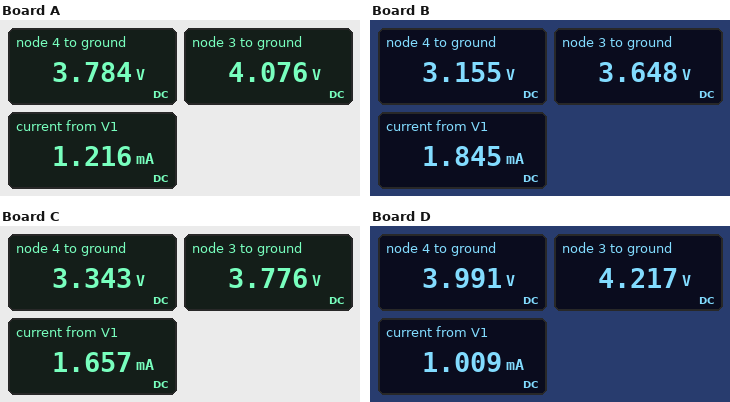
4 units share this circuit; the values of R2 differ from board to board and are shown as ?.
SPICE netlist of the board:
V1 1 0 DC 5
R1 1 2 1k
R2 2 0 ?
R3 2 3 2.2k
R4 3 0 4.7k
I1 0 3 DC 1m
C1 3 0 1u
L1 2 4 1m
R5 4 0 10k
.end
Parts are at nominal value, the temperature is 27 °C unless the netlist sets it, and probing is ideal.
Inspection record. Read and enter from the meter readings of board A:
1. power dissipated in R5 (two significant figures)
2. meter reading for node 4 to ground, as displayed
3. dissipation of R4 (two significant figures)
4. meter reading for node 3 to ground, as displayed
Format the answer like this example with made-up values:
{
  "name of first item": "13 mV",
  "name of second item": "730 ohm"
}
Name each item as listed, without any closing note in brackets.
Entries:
{
  "power dissipated in R5": "1.4 mW",
  "meter reading for node 4 to ground, as displayed": "3.784 V",
  "dissipation of R4": "3.5 mW",
  "meter reading for node 3 to ground, as displayed": "4.076 V"
}
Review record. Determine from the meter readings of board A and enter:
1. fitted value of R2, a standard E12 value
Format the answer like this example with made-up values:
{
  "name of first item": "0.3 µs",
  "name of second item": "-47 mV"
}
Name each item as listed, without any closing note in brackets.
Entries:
{
  "fitted value of R2, a standard E12 value": "3.9 kΩ"
}
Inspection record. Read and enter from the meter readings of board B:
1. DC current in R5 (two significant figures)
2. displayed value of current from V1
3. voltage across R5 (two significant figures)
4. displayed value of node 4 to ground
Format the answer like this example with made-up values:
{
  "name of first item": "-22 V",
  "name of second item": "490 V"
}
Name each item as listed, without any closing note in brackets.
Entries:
{
  "DC current in R5": "320 µA",
  "displayed value of current from V1": "1.845 mA",
  "voltage across R5": "3.2 V",
  "displayed value of node 4 to ground": "3.155 V"
}
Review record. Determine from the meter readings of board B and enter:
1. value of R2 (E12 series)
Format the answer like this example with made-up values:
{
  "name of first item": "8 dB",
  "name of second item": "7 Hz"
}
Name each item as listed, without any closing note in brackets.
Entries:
{
  "value of R2": "1.8 kΩ"
}
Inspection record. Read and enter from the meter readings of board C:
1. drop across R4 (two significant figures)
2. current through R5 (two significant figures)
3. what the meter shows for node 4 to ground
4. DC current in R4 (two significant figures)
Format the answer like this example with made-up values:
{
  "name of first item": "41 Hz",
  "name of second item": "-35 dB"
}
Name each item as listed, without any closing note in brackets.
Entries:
{
  "drop across R4": "3.8 V",
  "current through R5": "330 µA",
  "what the meter shows for node 4 to ground": "3.343 V",
  "DC current in R4": "800 µA"
}
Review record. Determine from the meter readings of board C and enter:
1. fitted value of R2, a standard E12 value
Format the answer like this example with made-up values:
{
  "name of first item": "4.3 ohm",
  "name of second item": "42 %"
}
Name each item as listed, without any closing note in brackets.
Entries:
{
  "fitted value of R2, a standard E12 value": "2.2 kΩ"
}
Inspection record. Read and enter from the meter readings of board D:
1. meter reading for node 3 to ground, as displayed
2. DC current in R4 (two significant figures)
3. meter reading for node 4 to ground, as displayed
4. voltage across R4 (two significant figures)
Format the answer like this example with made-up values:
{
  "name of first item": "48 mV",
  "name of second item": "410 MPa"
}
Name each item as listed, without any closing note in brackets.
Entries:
{
  "meter reading for node 3 to ground, as displayed": "4.217 V",
  "DC current in R4": "900 µA",
  "meter reading for node 4 to ground, as displayed": "3.991 V",
  "voltage across R4": "4.2 V"
}
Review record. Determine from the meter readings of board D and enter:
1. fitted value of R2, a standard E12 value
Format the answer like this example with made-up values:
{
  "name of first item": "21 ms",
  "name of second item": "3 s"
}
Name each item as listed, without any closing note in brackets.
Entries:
{
  "fitted value of R2, a standard E12 value": "5.6 kΩ"
}
